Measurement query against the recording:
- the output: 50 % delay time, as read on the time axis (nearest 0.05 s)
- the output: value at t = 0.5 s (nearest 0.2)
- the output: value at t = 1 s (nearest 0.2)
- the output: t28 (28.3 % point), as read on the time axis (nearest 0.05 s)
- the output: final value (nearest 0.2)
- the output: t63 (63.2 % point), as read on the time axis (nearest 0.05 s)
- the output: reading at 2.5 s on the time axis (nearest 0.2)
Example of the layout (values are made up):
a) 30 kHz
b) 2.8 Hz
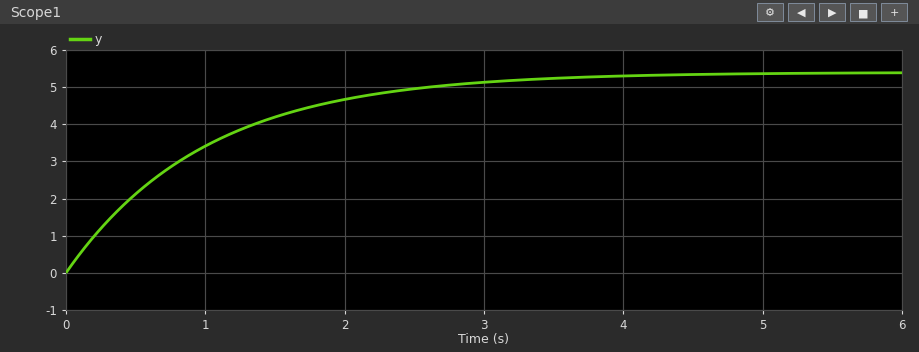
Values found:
a) 0.70 s
b) 2.2
c) 3.4
d) 0.35 s
e) 5.4
f) 1.00 s
g) 5.0
